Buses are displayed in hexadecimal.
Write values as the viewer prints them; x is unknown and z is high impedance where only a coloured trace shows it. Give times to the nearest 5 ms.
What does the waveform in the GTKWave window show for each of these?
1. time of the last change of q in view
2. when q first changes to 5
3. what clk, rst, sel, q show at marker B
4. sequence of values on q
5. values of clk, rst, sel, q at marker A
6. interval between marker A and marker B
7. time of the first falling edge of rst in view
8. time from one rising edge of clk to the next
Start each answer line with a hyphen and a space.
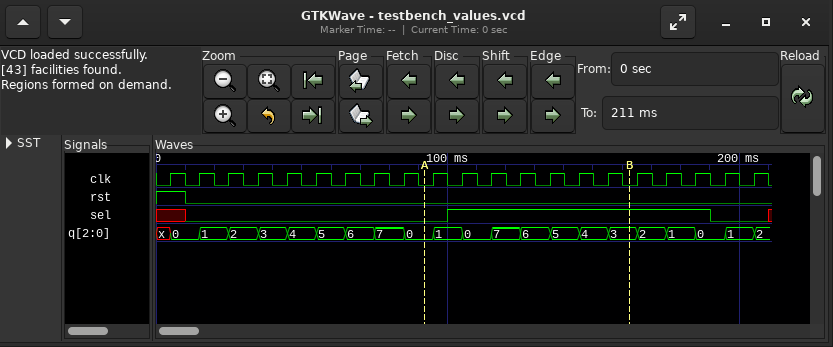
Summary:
- 205 ms
- 55 ms
- clk=0, rst=0, sel=1, q=3
- x, 0, 1, 2, 3, 4, 5, 6, 7, 0, 1, 0, 7, 6, 5, 4, 3, 2, 1, 0, 1, 2
- clk=0, rst=0, sel=0, q=0
- 70 ms
- 10 ms
- 10 ms
